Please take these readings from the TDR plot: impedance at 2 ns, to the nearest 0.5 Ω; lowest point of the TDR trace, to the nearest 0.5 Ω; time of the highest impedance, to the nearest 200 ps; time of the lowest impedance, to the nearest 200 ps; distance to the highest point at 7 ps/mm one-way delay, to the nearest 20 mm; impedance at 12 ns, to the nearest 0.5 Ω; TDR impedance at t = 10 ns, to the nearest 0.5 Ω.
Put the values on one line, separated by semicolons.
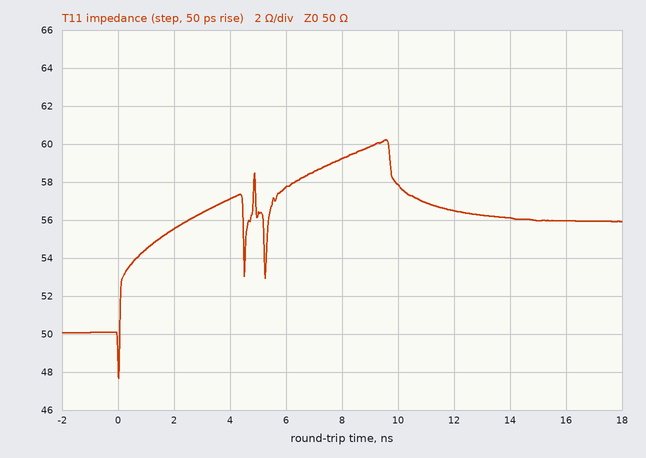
55.5 Ω; 47.5 Ω; 9.6 ns; 0.0 ns; 680 mm; 56.5 Ω; 58.0 Ω
